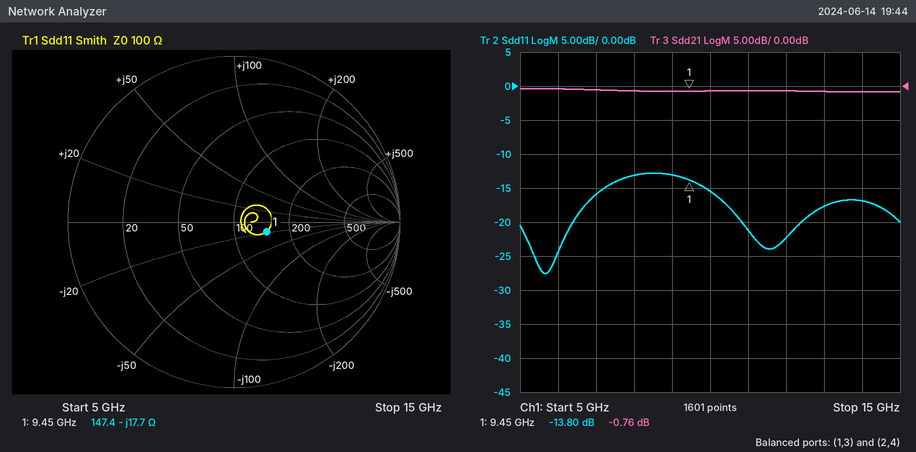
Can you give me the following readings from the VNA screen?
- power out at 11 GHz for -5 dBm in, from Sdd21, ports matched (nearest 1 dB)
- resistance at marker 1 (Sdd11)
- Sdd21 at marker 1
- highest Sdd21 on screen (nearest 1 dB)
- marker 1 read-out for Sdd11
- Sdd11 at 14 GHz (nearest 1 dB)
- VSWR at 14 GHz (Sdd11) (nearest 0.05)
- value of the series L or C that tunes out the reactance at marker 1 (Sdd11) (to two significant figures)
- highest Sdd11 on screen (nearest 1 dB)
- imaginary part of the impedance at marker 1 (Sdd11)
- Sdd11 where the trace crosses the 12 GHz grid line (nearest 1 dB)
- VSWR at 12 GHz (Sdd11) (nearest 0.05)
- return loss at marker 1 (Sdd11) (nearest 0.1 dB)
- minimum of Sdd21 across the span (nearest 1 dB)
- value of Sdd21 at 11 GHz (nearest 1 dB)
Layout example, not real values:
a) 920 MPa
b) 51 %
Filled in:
a) -6 dBm
b) 147.4 Ω
c) -0.76 dB
d) 0 dB
e) -13.80 dB
f) -17 dB
g) 1.35
h) 300 pH
i) -13 dB
j) -17.7 Ω
k) -22 dB
l) 1.15
m) 13.8 dB
n) -1 dB
o) -1 dB
